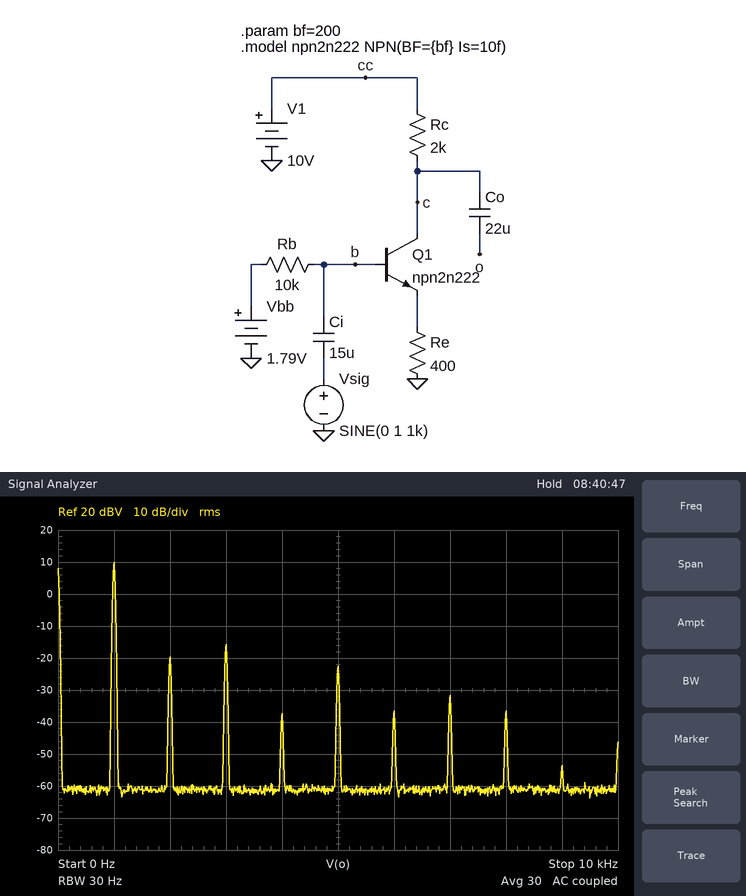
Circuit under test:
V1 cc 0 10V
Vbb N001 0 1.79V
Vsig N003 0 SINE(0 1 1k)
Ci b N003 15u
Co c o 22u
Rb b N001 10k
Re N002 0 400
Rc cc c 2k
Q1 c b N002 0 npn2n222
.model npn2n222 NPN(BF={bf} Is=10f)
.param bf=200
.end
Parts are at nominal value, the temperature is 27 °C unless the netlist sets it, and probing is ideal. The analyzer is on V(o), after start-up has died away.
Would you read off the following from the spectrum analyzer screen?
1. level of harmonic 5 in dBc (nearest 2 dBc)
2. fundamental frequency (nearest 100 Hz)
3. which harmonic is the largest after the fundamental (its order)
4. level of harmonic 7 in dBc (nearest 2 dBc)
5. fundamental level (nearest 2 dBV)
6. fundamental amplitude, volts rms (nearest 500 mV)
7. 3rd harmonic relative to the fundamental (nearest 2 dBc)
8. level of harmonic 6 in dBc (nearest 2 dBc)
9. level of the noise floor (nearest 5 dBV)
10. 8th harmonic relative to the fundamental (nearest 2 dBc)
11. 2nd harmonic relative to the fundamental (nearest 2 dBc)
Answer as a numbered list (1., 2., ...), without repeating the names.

1. -32 dBc
2. 1.0 kHz
3. 3
4. -42 dBc
5. 10 dBV
6. 3.0 V
7. -26 dBc
8. -46 dBc
9. -60 dBV
10. -46 dBc
11. -30 dBc
